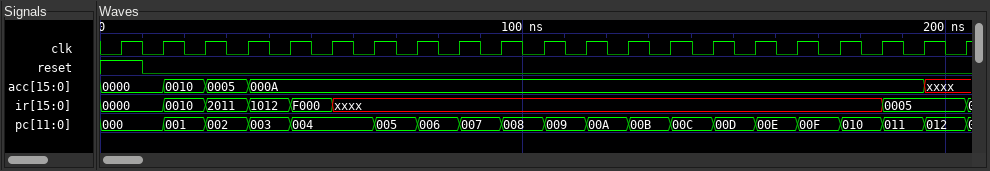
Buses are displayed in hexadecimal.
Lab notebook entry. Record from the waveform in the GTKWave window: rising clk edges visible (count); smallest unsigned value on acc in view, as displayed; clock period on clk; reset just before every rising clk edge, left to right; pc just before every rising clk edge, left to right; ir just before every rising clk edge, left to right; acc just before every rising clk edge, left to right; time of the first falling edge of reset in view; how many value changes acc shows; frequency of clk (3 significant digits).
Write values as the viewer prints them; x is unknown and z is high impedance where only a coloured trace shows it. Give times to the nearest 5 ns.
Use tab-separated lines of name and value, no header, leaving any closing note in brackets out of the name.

rising clk edges visible	21
smallest unsigned value on acc in view, as displayed	0000
clock period on clk	10 ns
reset just before every rising clk edge, left to right	1 0 0 0 0 0 0 0 0 0 0 0 0 0 0 0 0 0 0 0 0
pc just before every rising clk edge, left to right	000, 000, 001, 002, 003, 004, 004, 005, 006, 007, 008, 009, 00A, 00B, 00C, 00D, 00E, 00F, 010, 011, 012
ir just before every rising clk edge, left to right	0000, 0000, 0010, 2011, 1012, F000, xxxx, xxxx, xxxx, xxxx, xxxx, xxxx, xxxx, xxxx, xxxx, xxxx, xxxx, xxxx, xxxx, 0005, 0005
acc just before every rising clk edge, left to right	0000, 0000, 0010, 0005, 000A, 000A, 000A, 000A, 000A, 000A, 000A, 000A, 000A, 000A, 000A, 000A, 000A, 000A, 000A, 000A, xxxx
time of the first falling edge of reset in view	10 ns
how many value changes acc shows	4
frequency of clk	100 MHz
